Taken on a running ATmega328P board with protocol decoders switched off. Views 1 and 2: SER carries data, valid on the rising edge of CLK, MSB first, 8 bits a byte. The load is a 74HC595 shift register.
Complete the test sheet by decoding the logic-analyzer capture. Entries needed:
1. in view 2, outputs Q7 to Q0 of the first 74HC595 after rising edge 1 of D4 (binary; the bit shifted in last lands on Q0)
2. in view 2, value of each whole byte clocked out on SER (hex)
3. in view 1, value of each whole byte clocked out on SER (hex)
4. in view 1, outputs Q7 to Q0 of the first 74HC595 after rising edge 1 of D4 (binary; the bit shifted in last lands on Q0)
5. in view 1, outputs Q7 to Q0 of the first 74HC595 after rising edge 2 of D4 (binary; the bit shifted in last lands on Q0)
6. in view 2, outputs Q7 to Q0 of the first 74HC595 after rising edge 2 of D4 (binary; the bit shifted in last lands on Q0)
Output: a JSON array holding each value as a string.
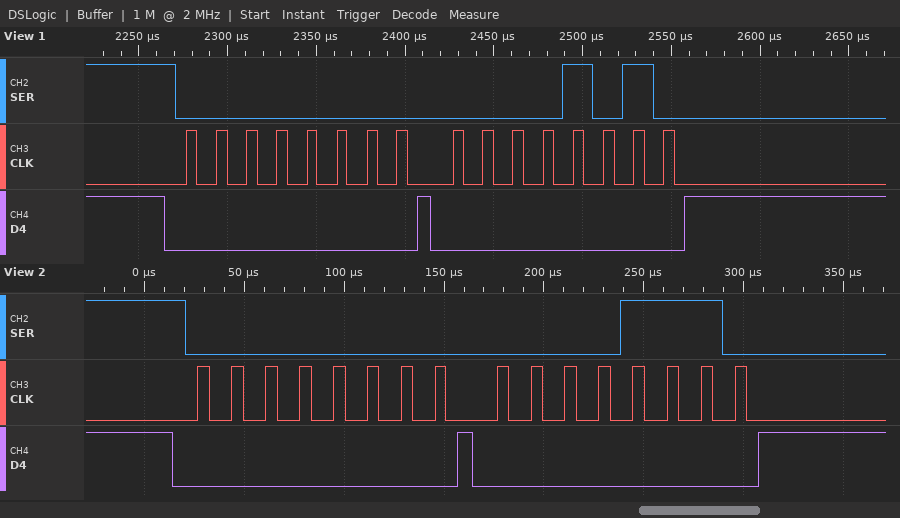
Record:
["00000000", "00 0E", "00 0A", "00000000", "00001010", "00001110"]
